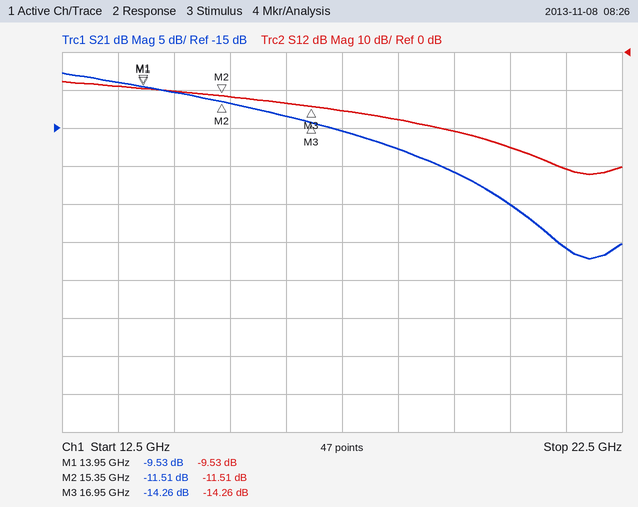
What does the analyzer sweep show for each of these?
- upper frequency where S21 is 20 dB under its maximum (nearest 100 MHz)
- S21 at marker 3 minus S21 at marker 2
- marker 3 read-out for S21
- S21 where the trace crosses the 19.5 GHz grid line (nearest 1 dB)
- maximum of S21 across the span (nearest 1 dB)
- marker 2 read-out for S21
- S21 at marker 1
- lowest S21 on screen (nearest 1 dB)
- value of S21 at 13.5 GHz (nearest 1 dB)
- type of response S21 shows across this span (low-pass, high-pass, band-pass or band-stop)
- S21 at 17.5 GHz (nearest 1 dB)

21.0 GHz
-2.75 dB
-14.26 dB
-21 dB
-8 dB
-11.51 dB
-9.53 dB
-32 dB
-9 dB
low-pass
-15 dB
